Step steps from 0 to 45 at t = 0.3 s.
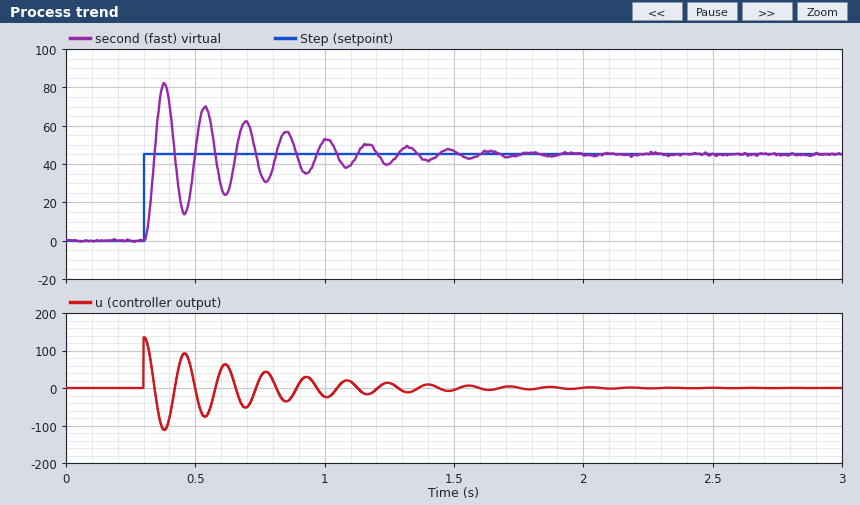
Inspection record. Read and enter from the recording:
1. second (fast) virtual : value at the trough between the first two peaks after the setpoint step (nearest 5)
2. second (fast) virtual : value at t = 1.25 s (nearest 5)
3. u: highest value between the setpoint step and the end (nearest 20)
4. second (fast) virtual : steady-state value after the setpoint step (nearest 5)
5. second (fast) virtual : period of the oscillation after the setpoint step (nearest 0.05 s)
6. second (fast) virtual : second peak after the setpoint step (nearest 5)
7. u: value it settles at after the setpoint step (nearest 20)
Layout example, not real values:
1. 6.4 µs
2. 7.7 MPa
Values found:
1. 15
2. 40
3. 140
4. 45
5. 0.15 s
6. 70
7. 0
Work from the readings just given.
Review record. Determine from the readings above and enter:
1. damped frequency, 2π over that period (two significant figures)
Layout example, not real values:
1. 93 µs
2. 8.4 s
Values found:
1. 42 rad/s
